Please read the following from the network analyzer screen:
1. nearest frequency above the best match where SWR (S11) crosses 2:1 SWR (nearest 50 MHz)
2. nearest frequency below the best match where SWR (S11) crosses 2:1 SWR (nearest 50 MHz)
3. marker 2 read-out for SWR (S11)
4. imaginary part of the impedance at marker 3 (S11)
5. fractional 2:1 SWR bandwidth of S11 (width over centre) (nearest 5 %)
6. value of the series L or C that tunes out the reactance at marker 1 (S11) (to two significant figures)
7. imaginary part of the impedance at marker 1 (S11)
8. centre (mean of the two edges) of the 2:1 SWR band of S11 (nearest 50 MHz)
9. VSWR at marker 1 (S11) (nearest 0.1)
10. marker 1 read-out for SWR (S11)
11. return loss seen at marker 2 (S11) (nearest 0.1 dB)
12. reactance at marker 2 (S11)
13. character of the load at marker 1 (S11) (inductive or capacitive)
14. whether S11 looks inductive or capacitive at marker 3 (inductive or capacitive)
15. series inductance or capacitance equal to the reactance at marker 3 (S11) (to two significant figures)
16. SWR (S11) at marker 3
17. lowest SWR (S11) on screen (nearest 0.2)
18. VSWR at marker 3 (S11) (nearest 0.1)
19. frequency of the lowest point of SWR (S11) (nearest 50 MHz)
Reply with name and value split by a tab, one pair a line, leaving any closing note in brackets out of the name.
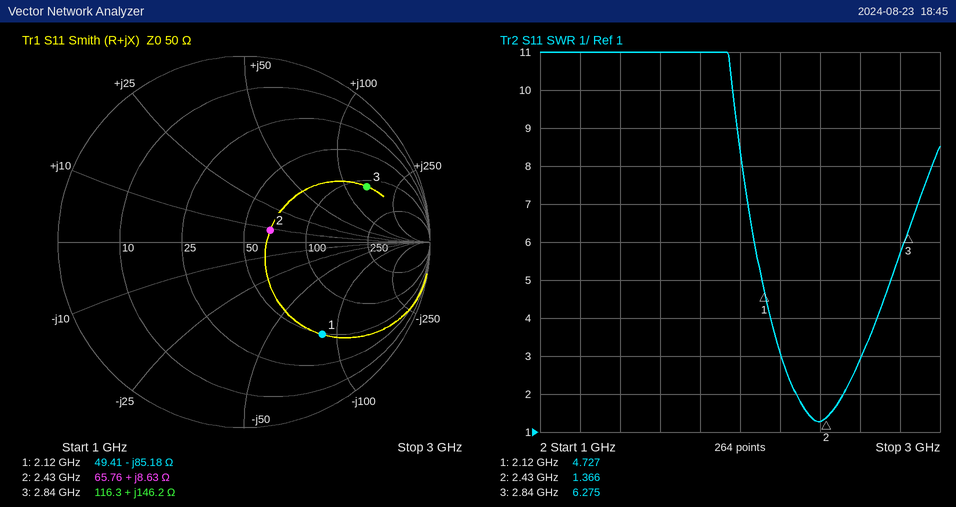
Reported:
nearest frequency above the best match where SWR (S11) crosses 2:1 SWR	2.50 GHz
nearest frequency below the best match where SWR (S11) crosses 2:1 SWR	2.30 GHz
marker 2 read-out for SWR	1.366
imaginary part of the impedance at marker 3	+146.2 Ω
fractional 2:1 SWR bandwidth of S11 (width over centre)	10 %
value of the series L or C that tunes out the reactance at marker 1 (S11)	6.4 nH
imaginary part of the impedance at marker 1	-85.18 Ω
centre (mean of the two edges) of the 2:1 SWR band of S11	2.40 GHz
VSWR at marker 1 (S11)	4.7
marker 1 read-out for SWR	4.727
return loss seen at marker 2 (S11)	16.2 dB
reactance at marker 2	+8.63 Ω
character of the load at marker 1 (S11)	capacitive
whether S11 looks inductive or capacitive at marker 3	inductive
series inductance or capacitance equal to the reactance at marker 3 (S11)	8.2 nH
SWR (S11) at marker 3	6.275
lowest SWR (S11) on screen	1.2
VSWR at marker 3 (S11)	6.3
frequency of the lowest point of SWR (S11)	2.40 GHz
